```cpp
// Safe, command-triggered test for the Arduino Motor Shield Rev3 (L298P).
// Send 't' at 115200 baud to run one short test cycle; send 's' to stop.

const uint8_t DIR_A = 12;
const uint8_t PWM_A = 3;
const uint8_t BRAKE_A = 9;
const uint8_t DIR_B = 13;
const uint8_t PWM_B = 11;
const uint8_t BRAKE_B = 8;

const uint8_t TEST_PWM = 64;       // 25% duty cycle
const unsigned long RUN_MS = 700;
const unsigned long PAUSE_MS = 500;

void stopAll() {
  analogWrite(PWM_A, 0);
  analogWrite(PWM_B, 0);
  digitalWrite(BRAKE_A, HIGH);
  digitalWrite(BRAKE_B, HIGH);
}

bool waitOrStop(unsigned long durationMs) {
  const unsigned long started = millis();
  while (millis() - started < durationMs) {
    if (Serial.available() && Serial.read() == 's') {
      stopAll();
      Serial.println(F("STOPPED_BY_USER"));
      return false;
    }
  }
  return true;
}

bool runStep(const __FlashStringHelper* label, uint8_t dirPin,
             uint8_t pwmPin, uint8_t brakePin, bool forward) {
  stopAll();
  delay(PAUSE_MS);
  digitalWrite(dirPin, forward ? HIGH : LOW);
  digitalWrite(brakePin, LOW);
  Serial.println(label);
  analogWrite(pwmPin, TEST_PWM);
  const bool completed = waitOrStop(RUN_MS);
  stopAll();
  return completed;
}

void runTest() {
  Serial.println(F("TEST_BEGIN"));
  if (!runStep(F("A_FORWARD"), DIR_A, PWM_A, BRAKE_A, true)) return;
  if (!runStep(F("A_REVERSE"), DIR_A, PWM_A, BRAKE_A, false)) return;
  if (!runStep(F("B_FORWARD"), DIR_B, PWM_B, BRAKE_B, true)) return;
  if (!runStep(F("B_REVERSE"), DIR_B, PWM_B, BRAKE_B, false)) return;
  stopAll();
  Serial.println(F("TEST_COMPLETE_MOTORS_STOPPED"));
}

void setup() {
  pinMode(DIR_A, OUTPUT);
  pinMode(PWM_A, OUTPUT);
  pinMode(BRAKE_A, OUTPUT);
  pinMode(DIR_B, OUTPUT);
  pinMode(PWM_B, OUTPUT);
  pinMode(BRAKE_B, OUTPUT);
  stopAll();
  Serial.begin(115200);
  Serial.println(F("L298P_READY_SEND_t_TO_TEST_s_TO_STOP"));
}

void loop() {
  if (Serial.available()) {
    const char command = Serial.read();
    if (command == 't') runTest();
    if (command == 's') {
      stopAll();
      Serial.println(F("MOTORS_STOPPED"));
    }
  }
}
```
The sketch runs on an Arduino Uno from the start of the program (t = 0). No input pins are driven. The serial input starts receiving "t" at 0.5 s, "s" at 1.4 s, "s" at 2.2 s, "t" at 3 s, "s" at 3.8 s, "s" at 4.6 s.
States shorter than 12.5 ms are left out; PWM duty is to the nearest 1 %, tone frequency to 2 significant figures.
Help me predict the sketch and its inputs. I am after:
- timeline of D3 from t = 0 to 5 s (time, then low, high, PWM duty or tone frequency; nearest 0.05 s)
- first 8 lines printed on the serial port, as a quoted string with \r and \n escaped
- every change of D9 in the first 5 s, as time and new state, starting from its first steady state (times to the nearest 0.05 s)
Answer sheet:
0 s low; 1 s PWM 25 %; 1.4 s low; 3.5 s PWM 25 %; 3.8 s low
"L298P_READY_SEND_t_TO_TEST_s_TO_STOP\r\nTEST_BEGIN\r\nA_FORWARD\r\nSTOPPED_BY_USER\r\nMOTORS_STOPPED\r\nTEST_BEGIN\r\nA_FORWARD\r\nSTOPPED_BY_USER\r\n"
0 s high; 1 s low; 1.4 s high; 3.5 s low; 3.8 s high
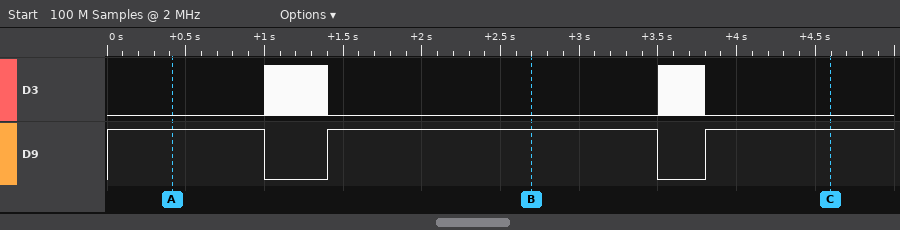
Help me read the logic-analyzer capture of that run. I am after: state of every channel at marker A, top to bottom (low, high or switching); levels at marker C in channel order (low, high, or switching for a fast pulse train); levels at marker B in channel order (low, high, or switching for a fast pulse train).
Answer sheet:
D3 low, D9 high
D3 low, D9 high
D3 low, D9 high
